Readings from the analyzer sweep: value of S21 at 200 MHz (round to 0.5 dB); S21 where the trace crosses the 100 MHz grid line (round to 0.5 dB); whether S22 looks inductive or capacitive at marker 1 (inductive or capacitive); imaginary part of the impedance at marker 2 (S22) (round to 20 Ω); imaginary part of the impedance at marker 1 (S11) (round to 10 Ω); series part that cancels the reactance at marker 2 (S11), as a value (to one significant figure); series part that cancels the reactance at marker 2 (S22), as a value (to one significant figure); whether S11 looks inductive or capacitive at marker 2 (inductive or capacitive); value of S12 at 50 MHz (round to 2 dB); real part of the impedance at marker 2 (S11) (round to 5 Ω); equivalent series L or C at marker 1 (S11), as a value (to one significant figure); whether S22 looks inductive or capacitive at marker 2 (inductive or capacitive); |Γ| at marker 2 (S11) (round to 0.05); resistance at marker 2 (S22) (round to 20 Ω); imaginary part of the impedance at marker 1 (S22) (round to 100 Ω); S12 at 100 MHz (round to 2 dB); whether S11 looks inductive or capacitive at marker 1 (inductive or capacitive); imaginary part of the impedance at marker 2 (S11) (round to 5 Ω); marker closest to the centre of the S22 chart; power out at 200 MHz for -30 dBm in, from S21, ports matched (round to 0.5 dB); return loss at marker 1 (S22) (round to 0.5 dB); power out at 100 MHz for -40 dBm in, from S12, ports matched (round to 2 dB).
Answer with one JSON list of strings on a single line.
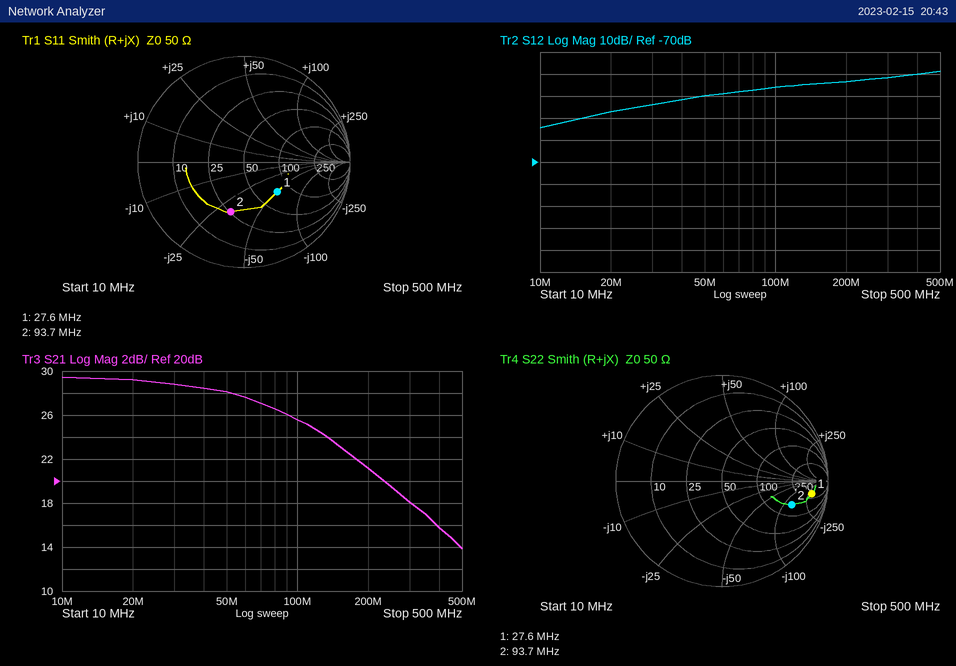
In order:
["21.0 dB", "25.5 dB", "capacitive", "-140 Ω", "-50 Ω", "50 nH", "200 nH", "capacitive", "-40 dB", "25 Ω", "100 pF", "capacitive", "0.50", "160 Ω", "-300 Ω", "-36 dB", "capacitive", "-30 Ω", "marker 2", "-9.0 dBm", "1.5 dB", "-76 dBm"]
